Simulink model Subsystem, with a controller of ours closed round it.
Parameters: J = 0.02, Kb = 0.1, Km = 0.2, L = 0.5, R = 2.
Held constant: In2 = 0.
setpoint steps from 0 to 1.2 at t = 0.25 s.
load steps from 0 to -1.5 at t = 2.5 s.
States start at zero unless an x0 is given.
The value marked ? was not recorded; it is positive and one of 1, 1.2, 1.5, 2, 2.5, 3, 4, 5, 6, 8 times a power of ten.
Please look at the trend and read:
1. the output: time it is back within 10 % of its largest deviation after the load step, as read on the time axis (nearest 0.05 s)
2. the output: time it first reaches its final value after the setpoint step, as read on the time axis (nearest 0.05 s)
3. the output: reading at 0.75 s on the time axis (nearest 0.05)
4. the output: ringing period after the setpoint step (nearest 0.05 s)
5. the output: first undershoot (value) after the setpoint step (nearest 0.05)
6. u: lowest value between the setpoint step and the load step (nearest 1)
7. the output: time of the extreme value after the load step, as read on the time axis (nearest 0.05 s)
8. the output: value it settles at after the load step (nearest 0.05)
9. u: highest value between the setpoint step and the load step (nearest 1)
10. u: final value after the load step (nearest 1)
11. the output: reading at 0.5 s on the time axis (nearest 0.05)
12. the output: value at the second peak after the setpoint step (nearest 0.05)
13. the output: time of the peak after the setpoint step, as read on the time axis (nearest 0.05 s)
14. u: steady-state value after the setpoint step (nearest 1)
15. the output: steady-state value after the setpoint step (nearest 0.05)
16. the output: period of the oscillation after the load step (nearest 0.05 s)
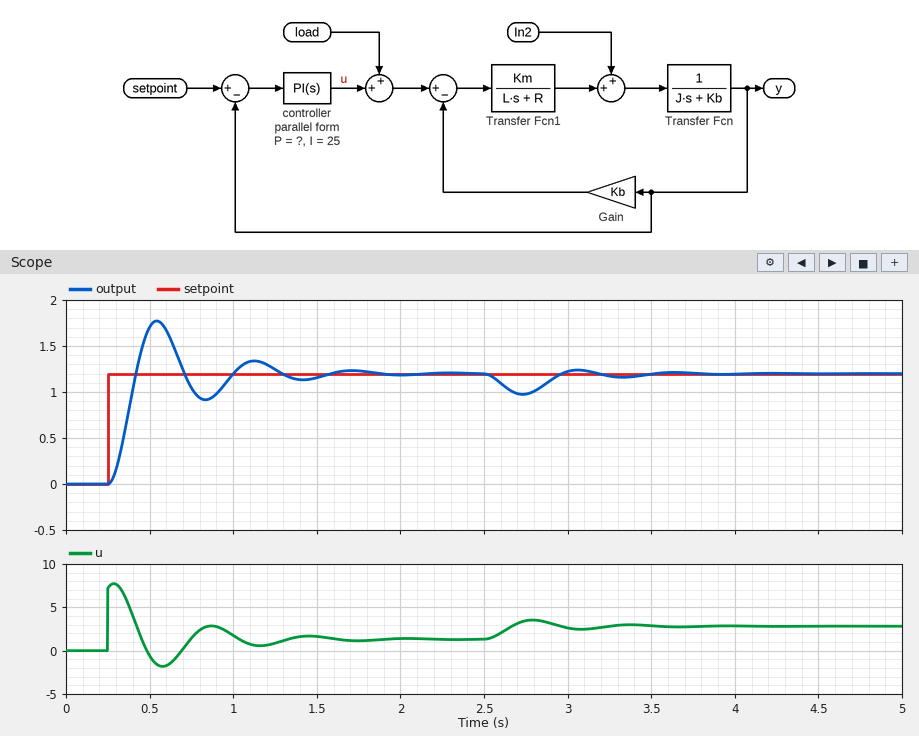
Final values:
3.45 s
0.40 s
1.05
0.60 s
0.90
-2
2.75 s
1.20
8
3
1.70
1.35
0.55 s
1
1.20
0.60 s
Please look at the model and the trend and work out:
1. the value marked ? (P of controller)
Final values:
6
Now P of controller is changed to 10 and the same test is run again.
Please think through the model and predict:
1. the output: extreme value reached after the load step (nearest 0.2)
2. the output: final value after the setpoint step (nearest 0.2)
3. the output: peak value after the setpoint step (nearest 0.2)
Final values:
1.0
1.2
1.8
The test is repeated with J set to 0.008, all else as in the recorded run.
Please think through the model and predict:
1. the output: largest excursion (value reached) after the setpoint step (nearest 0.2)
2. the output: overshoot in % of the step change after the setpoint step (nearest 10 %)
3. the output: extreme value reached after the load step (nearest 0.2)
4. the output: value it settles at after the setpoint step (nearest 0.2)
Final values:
1.6
30 %
1.0
1.2
